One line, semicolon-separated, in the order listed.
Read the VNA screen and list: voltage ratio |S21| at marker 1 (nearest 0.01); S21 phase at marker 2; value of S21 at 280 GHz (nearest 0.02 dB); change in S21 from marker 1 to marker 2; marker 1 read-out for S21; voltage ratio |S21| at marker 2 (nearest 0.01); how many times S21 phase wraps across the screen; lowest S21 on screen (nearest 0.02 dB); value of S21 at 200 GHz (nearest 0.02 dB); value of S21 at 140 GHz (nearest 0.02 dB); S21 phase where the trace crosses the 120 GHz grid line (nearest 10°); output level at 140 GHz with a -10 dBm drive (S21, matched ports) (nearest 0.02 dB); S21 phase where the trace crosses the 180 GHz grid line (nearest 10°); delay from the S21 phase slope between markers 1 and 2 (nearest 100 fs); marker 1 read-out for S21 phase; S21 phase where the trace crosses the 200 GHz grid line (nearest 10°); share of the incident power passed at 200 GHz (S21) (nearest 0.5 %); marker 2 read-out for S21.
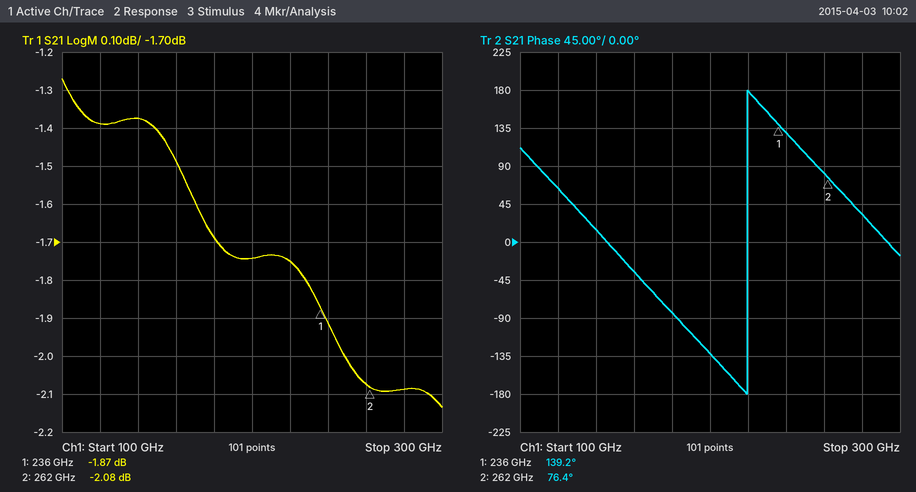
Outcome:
0.81; 76.4°; -2.08 dB; -0.21 dB; -1.87 dB; 0.79; 1; -2.14 dB; -1.74 dB; -1.38 dB; 60°; -11.38 dBm; -80°; 6.7 ps; 139.2°; -130°; 67.0 %; -2.08 dB
